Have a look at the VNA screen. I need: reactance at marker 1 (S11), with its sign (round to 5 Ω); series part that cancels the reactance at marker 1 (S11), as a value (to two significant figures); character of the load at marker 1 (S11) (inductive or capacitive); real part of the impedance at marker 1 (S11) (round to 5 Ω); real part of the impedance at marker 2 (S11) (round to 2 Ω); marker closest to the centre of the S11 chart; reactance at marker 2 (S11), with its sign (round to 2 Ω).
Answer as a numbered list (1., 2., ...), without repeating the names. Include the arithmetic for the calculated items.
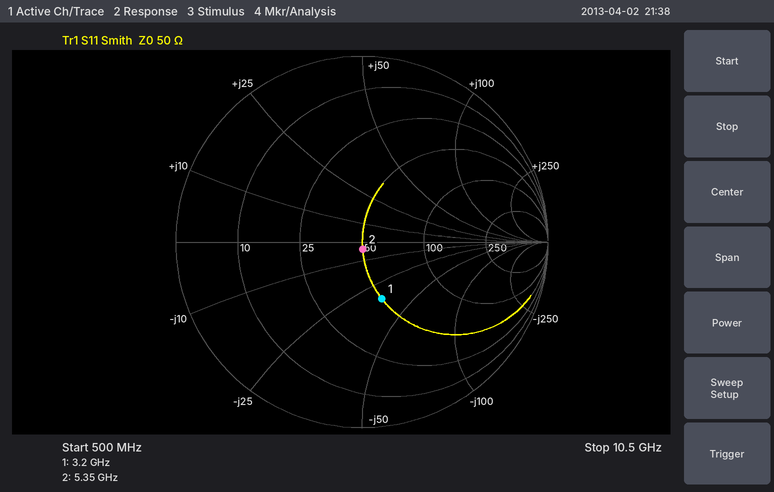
1. -35 Ω
2. L = 35 Ω/(2π × 3.2 GHz) ≈ 1.7 nH
3. capacitive
4. 50 Ω
5. 50 Ω
6. marker 2
7. -4 Ω
